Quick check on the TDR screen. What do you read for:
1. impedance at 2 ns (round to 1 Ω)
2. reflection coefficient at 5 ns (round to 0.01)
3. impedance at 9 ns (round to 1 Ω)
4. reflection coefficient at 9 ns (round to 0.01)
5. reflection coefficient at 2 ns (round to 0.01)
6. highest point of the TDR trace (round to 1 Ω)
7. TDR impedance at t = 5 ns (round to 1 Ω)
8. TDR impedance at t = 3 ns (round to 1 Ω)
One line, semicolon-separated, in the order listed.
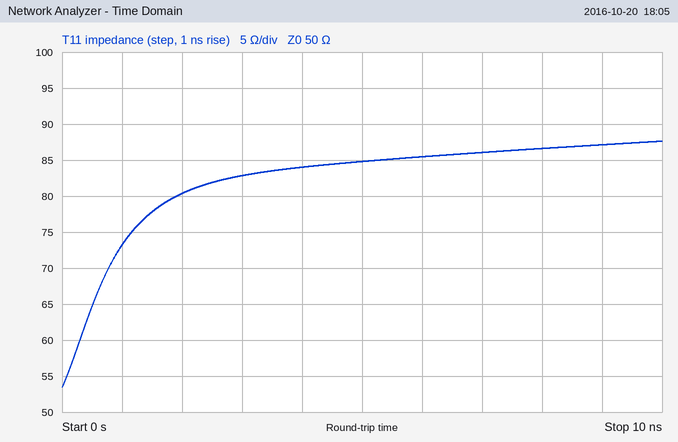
80 Ω; +0.26; 87 Ω; +0.27; +0.23; 88 Ω; 85 Ω; 83 Ω
